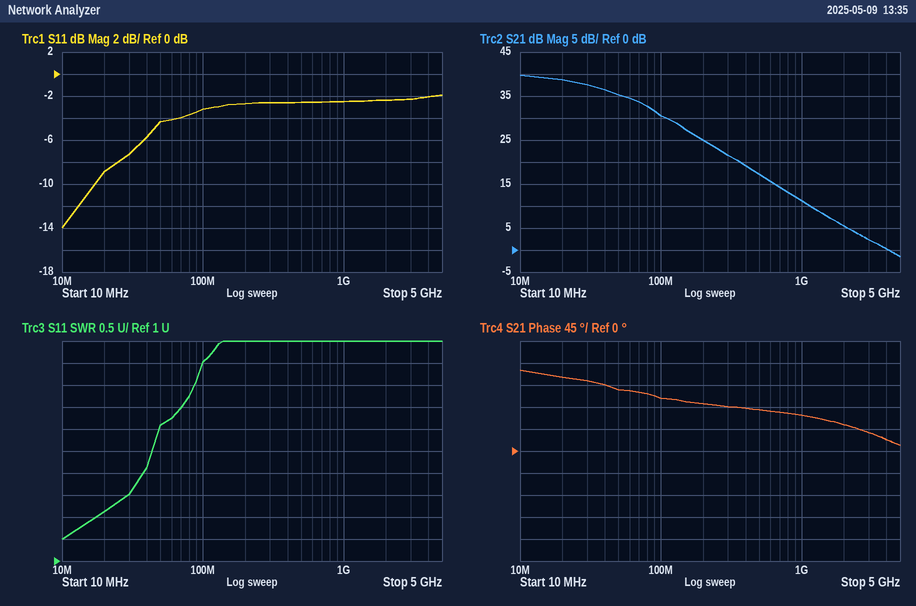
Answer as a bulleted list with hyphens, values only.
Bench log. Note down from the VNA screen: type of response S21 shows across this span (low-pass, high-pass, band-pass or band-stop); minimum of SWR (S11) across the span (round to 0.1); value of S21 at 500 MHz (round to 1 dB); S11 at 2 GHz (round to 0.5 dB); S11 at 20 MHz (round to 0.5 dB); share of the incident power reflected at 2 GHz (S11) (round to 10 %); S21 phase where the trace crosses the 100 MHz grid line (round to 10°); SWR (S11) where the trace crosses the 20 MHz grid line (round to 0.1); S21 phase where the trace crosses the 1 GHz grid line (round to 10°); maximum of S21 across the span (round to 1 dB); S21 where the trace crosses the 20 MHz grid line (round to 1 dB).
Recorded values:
- low-pass
- 1.5
- 17 dB
- -2.5 dB
- -9.0 dB
- 60 %
- 110°
- 2.1
- 70°
- 40 dB
- 39 dB
